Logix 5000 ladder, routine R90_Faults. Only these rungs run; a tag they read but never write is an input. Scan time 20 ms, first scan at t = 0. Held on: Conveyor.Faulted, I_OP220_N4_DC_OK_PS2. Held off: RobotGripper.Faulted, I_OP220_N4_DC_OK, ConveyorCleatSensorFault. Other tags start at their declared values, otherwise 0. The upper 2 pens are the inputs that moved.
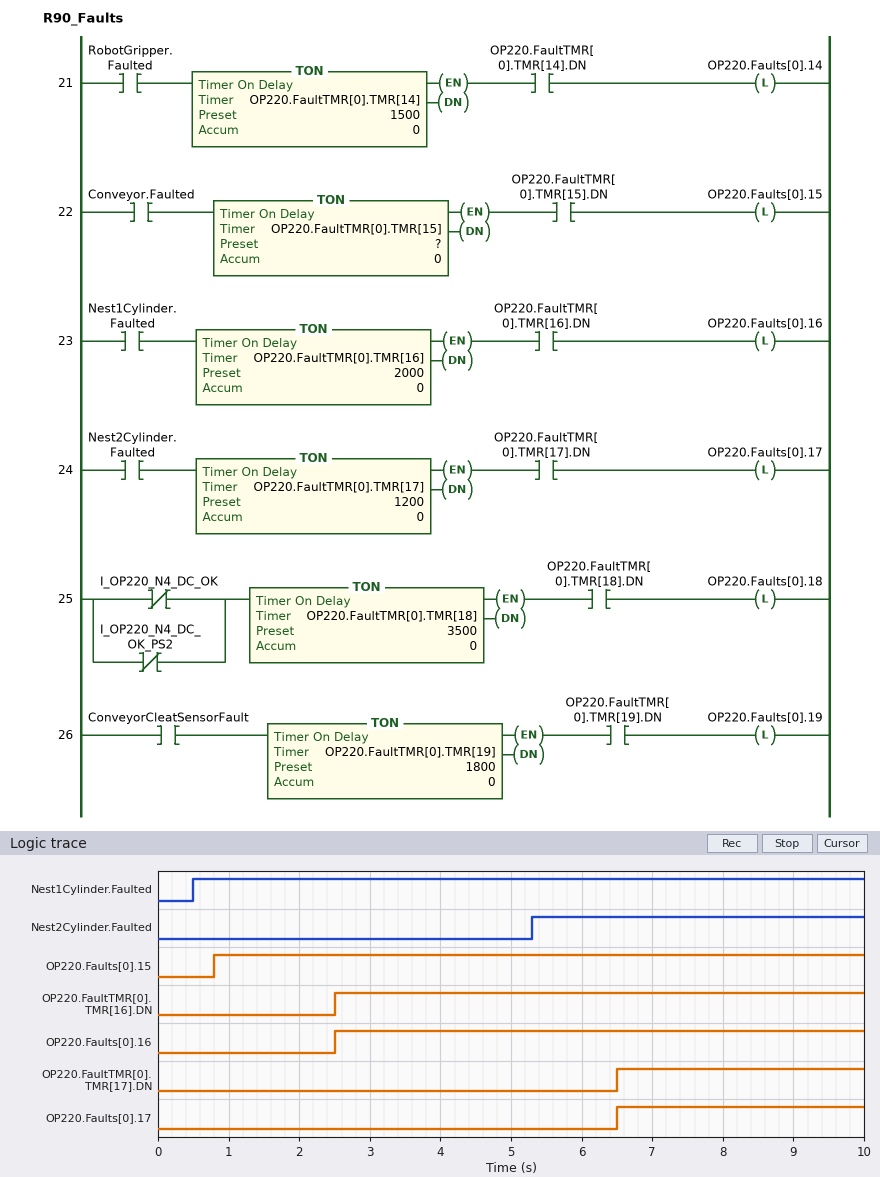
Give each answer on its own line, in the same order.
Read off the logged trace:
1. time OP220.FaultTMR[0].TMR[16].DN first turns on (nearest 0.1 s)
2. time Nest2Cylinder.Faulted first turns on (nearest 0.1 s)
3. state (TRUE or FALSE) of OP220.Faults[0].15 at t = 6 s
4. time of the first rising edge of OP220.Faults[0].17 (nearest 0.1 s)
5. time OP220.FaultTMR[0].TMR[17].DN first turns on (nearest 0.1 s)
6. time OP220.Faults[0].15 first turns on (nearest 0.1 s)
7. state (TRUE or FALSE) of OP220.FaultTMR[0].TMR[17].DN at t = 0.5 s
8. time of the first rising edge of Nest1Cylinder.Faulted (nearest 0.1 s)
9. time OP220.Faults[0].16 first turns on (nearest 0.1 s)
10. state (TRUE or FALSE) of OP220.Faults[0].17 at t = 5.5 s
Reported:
2.5 s
5.3 s
TRUE
6.5 s
6.5 s
0.8 s
FALSE
0.5 s
2.5 s
FALSE
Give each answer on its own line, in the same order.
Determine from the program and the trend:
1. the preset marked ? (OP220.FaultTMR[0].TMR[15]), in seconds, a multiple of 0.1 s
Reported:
0.8 s
